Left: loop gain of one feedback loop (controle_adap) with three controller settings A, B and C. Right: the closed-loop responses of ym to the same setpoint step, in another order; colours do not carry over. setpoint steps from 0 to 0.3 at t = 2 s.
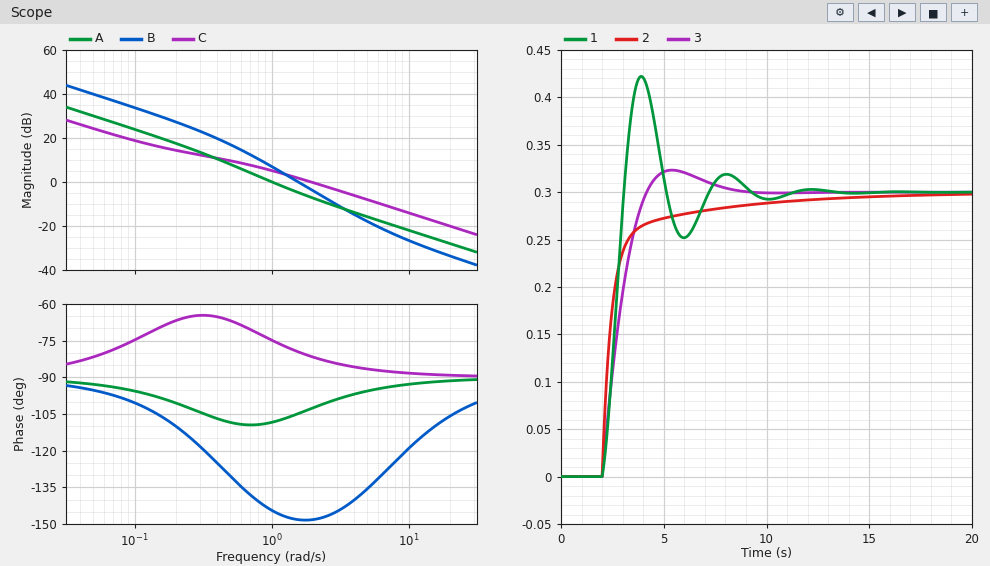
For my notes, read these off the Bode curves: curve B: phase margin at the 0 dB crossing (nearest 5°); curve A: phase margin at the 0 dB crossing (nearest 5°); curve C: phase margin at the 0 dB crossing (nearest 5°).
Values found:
30°
70°
100°
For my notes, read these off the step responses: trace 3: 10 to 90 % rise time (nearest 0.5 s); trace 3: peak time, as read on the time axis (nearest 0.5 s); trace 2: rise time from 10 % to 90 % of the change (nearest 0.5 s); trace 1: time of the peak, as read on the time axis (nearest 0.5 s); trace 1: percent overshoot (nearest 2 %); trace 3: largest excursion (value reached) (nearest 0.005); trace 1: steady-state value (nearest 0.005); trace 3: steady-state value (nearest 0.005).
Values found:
1.5 s
5.5 s
2.5 s
4.0 s
40 %
0.325
0.300
0.300
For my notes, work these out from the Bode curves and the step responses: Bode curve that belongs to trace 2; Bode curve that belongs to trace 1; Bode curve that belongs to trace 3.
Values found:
C
B
A
